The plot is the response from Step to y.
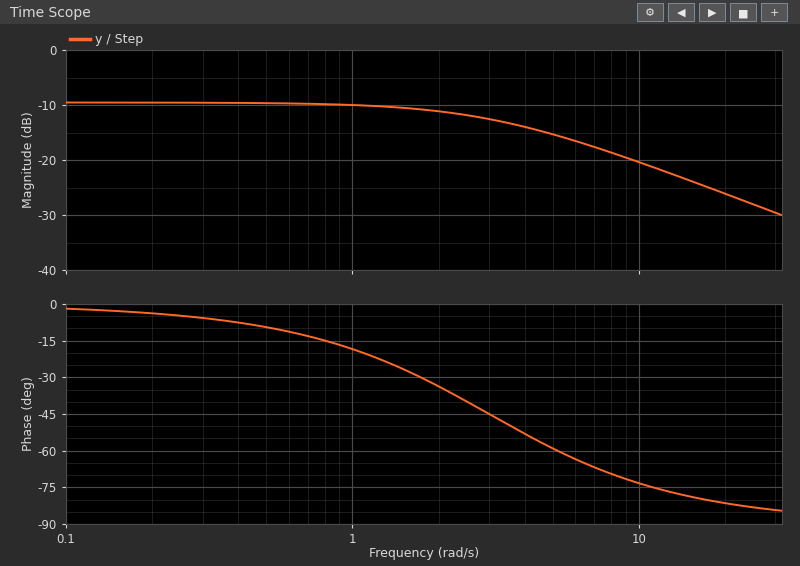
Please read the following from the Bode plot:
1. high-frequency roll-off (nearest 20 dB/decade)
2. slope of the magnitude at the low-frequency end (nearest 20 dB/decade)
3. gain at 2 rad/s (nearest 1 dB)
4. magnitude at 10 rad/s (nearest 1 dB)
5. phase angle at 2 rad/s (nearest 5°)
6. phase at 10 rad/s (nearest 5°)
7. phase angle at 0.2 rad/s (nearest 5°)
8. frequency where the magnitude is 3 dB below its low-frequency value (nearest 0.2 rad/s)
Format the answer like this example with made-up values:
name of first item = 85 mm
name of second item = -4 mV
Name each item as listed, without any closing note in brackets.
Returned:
high-frequency roll-off = -20 dB/decade
slope of the magnitude at the low-frequency end = 0 dB/decade
gain at 2 rad/s = -11 dB
magnitude at 10 rad/s = -20 dB
phase angle at 2 rad/s = -35°
phase at 10 rad/s = -75°
phase angle at 0.2 rad/s = -5°
frequency where the magnitude is 3 dB below its low-frequency value = 3.0 rad/s
